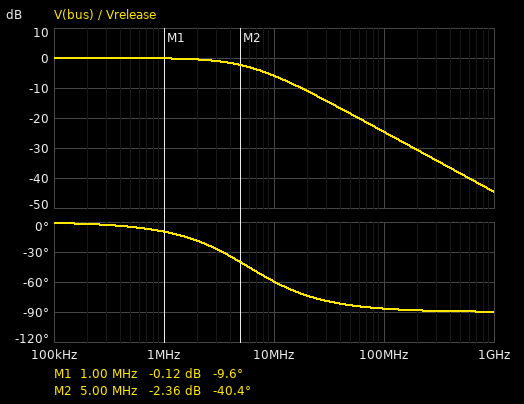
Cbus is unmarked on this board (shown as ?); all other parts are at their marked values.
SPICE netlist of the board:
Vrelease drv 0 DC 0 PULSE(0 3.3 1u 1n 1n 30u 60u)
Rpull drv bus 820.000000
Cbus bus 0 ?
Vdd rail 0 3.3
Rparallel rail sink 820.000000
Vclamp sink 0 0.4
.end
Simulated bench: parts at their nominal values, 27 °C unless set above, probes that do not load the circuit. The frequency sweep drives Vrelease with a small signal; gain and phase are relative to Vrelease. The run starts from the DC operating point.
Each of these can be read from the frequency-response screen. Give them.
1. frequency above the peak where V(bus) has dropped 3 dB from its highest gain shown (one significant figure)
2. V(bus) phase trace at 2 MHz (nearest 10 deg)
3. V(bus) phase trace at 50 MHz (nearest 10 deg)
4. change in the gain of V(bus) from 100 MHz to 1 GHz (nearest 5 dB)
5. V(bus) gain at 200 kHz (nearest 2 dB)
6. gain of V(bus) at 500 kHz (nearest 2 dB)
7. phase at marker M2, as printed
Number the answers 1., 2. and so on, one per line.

1. 6 MHz
2. -20 deg
3. -80 deg
4. -20 dB
5. 0 dB
6. 0 dB
7. -40.4 deg
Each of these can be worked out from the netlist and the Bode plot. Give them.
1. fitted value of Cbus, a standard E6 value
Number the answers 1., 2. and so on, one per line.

1. 33 pF
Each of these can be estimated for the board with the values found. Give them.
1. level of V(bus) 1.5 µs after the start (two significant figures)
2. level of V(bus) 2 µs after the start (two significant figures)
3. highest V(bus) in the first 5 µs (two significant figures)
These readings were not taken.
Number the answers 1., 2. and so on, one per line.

1. 3.3 V
2. 3.3 V
3. 3.3 V
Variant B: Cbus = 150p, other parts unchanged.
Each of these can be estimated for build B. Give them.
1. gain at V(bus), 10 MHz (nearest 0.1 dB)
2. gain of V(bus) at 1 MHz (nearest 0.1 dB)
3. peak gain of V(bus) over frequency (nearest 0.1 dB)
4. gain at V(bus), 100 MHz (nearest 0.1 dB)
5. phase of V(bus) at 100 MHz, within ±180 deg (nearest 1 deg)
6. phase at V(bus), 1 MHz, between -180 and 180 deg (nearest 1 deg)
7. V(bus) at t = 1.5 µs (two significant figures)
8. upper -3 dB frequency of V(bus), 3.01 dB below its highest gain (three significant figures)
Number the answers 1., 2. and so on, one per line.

1. -17.8 dB
2. -2.0 dB
3. 0 dB
4. -37.8 dB
5. -89 deg
6. -38 deg
7. 3.2 V
8. 1.29 MHz
